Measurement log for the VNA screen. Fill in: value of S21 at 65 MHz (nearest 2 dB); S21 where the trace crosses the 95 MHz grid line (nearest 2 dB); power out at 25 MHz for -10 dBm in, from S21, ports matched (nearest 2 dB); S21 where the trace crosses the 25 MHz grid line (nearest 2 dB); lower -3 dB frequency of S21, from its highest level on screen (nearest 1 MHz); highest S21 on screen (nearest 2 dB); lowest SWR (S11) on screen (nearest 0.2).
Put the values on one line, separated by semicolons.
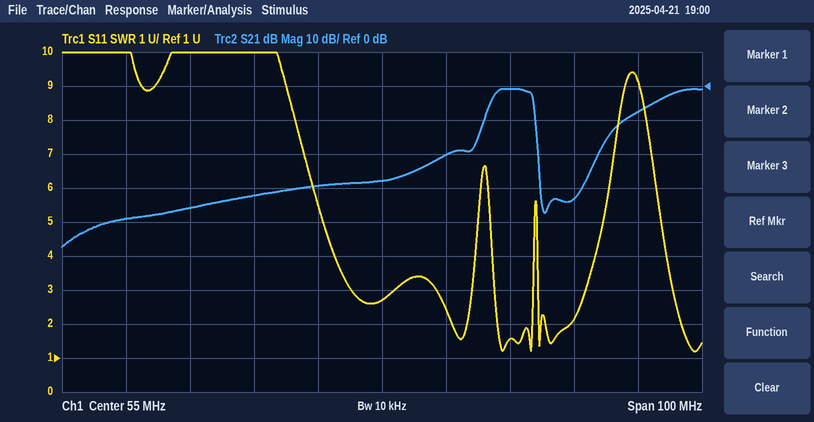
-20 dB; -8 dB; -46 dBm; -36 dB; 72 MHz; 0 dB; 1.2
